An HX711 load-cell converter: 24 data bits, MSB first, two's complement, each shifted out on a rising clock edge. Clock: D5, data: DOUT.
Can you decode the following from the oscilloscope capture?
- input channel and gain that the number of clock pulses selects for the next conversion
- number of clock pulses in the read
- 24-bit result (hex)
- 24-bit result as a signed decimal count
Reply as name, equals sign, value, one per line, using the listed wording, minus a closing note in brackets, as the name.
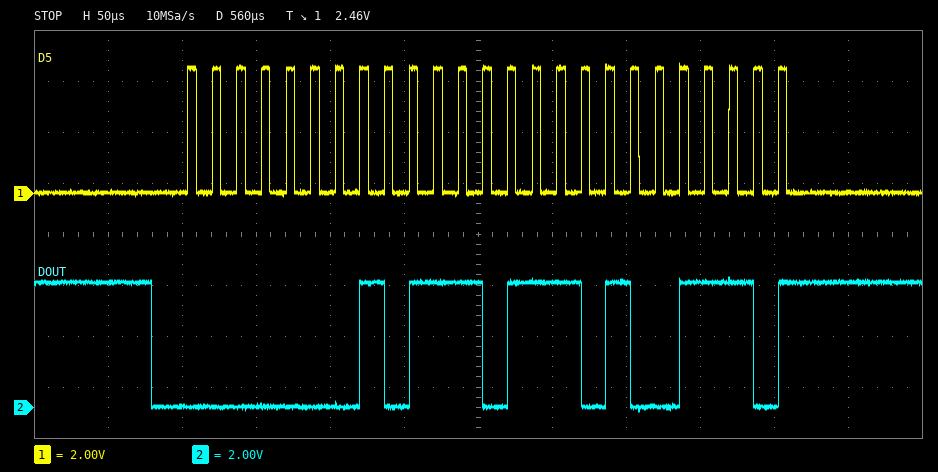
input channel and gain that the number of clock pulses selects for the next conversion = channel A, gain 128
number of clock pulses in the read = 25
24-bit result = 0x01774E
24-bit result as a signed decimal count = 96078
